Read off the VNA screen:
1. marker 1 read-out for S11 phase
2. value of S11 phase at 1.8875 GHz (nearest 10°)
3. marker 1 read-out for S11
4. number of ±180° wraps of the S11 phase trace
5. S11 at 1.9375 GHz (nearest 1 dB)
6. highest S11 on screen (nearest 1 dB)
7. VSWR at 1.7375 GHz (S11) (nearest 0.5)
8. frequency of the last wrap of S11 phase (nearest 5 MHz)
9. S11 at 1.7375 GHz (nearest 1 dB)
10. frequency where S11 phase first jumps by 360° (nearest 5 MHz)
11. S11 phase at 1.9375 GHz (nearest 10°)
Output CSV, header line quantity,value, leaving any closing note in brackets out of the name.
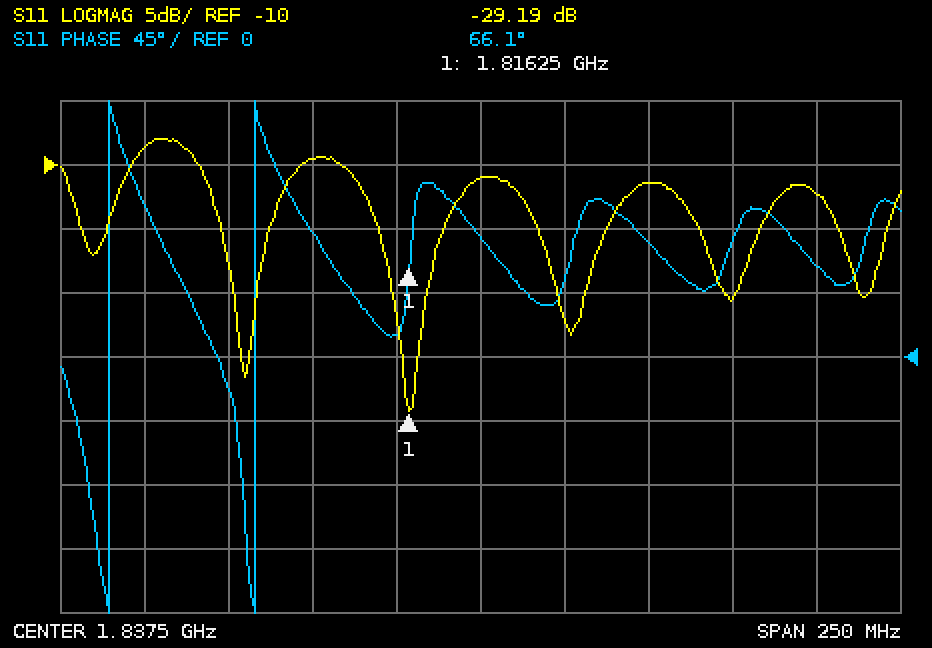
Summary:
quantity,value
marker 1 read-out for S11 phase,66.1°
value of S11 phase at 1.8875 GHz,80°
marker 1 read-out for S11,-29.19 dB
number of ±180° wraps of the S11 phase trace,2
S11 at 1.9375 GHz,-12 dB
highest S11 on screen,-8 dB
VSWR at 1.7375 GHz (S11),2.0
frequency of the last wrap of S11 phase,1.770 GHz
S11 at 1.7375 GHz,-9 dB
frequency where S11 phase first jumps by 360°,1.725 GHz
S11 phase at 1.9375 GHz,60°
